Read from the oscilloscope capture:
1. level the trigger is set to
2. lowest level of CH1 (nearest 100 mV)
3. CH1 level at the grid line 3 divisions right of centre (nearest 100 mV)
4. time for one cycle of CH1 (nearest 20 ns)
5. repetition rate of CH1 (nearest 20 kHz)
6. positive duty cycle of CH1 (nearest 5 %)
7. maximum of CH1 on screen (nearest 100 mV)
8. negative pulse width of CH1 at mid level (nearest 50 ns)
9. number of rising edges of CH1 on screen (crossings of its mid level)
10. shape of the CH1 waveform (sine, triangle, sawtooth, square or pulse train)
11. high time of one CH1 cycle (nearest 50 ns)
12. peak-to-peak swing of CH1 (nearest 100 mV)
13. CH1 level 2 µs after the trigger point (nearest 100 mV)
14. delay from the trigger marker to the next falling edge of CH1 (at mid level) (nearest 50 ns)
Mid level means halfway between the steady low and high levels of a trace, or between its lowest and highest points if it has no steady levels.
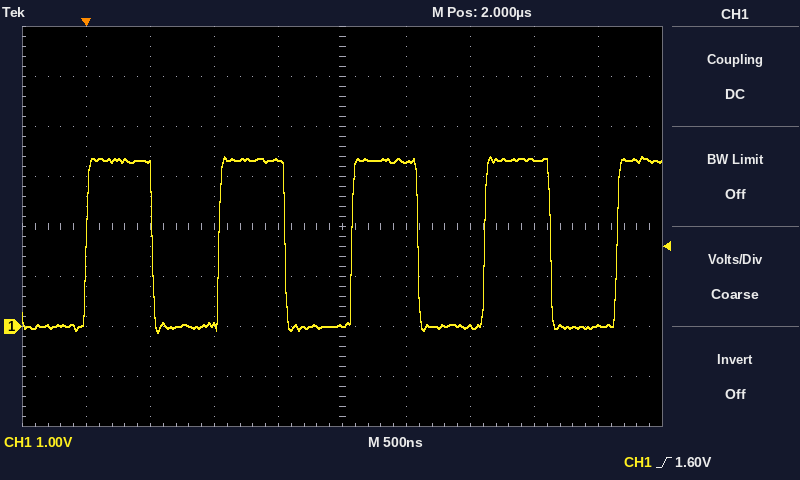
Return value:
1.60 V
-100 mV
3.3 V
1.04 µs
960 kHz
50 %
3.4 V
500 ns
5
square
500 ns
3.5 V
0.0 V
500 ns
